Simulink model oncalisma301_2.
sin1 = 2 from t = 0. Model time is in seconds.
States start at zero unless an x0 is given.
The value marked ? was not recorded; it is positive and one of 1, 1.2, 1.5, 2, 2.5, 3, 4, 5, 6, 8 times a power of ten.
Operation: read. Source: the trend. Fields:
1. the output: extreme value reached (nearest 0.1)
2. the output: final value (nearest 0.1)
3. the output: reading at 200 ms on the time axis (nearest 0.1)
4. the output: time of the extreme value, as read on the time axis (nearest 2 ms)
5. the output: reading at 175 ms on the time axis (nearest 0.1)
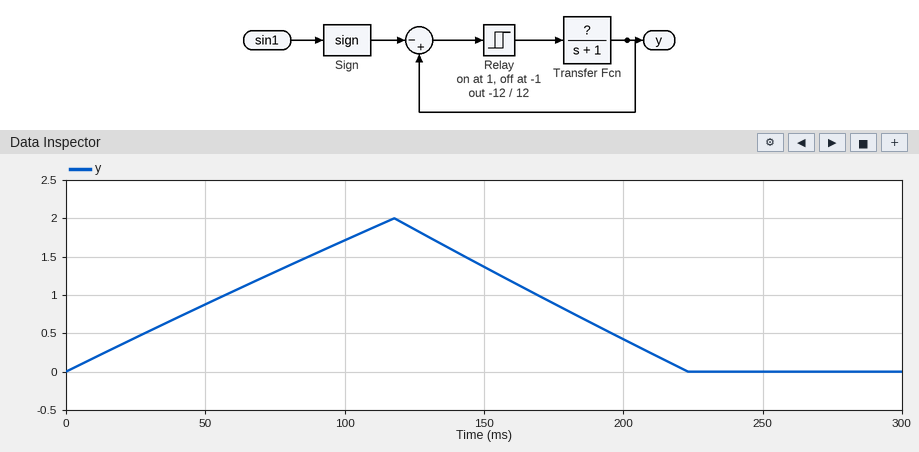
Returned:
2.0
0.0
0.4
118 ms
0.9
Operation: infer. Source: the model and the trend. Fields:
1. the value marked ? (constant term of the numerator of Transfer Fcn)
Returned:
1.5
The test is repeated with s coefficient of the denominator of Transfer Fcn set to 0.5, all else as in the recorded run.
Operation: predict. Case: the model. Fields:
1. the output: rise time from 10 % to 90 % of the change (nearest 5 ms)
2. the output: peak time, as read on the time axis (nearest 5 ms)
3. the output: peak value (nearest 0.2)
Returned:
20 ms
60 ms
2.0
